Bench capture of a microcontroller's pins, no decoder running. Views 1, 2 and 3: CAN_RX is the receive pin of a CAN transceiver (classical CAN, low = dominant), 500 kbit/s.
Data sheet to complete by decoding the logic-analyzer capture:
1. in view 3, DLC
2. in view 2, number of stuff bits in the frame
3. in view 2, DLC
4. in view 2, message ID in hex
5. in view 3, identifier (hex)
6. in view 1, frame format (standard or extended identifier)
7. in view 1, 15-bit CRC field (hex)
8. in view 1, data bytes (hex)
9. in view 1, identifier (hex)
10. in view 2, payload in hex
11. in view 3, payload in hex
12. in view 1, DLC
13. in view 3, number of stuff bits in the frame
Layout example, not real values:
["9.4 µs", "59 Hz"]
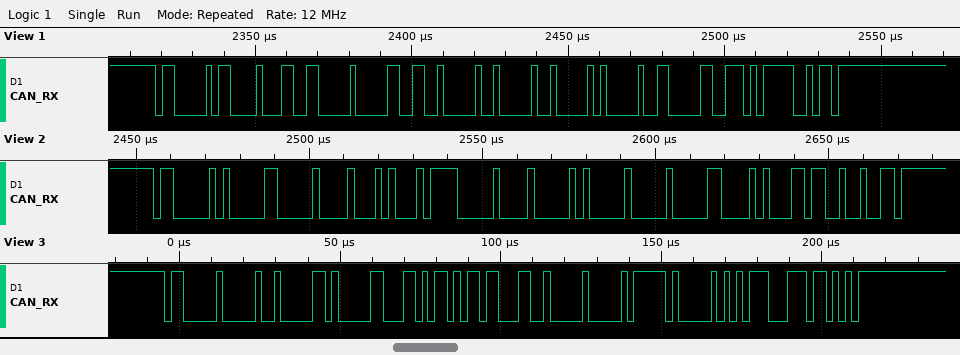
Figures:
["8", "8", "8", "0x604", "0x600", "standard", "0x75F5", "CC 00 99 01 01 02 03 04", "0x606", "02 28 BC 01 02 00 02 14", "28 23 5A D8 C8 00 FC 0A", "8", "8"]
